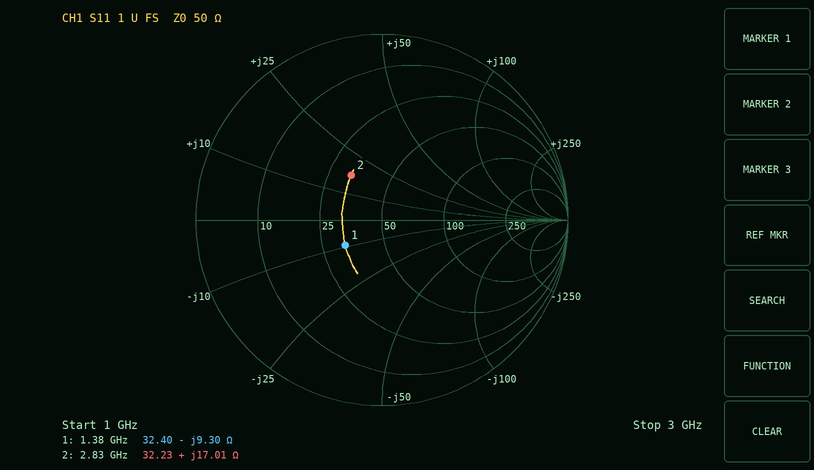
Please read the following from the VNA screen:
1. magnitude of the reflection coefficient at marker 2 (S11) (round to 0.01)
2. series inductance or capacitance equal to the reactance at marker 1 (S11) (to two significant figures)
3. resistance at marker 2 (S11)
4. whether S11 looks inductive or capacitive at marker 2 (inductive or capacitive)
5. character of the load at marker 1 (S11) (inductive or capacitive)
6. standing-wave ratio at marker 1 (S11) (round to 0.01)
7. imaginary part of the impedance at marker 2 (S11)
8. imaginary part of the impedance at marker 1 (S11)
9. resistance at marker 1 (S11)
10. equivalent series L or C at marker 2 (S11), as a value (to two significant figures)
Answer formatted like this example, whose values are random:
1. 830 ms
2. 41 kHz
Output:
1. 0.29
2. 12 pF
3. 32.23 Ω
4. inductive
5. capacitive
6. 1.63
7. +17.01 Ω
8. -9.30 Ω
9. 32.40 Ω
10. 960 pH
